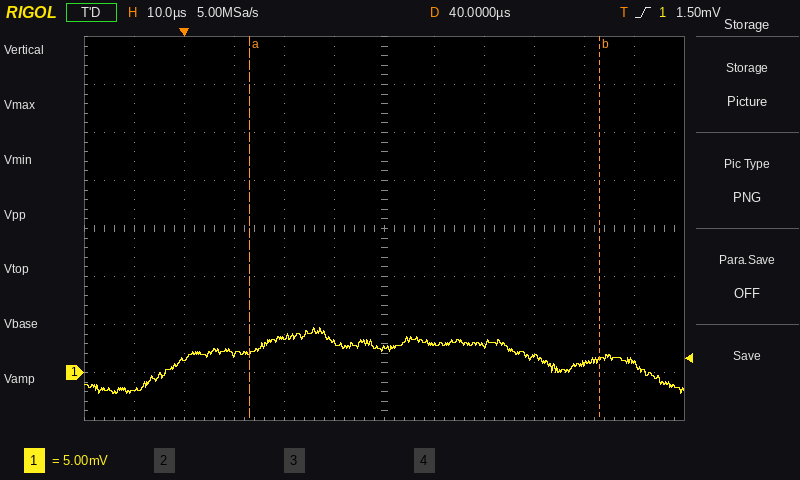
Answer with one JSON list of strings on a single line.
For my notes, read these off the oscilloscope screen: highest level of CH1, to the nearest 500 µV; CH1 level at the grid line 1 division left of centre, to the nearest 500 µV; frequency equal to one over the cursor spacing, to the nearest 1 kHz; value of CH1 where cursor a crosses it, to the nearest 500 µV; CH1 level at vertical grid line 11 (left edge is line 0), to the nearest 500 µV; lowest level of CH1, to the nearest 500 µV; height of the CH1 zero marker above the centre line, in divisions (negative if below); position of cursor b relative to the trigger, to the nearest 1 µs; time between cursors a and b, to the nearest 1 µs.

["4.5 mV", "3.0 mV", "14 kHz", "2.0 mV", "1.0 mV", "-2.0 mV", "-3.0 div", "+83 µs", "70 µs"]
